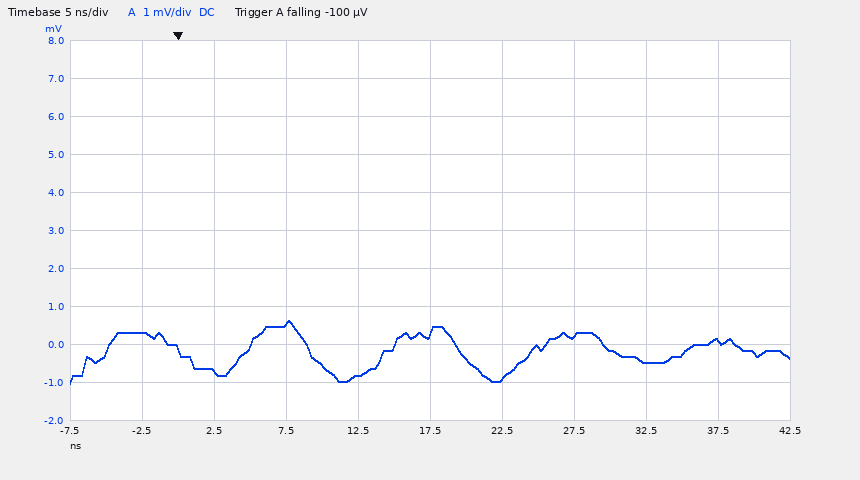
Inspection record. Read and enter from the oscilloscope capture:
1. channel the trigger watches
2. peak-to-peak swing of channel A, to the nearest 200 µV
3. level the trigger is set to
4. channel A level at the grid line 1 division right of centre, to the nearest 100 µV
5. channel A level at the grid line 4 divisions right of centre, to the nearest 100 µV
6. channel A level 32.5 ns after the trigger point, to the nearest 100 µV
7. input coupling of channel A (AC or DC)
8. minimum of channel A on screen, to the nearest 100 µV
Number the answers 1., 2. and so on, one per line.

1. channel A
2. 1.6 mV
3. -100 µV
4. -900 µV
5. 100 µV
6. -500 µV
7. DC
8. -1.0 mV
